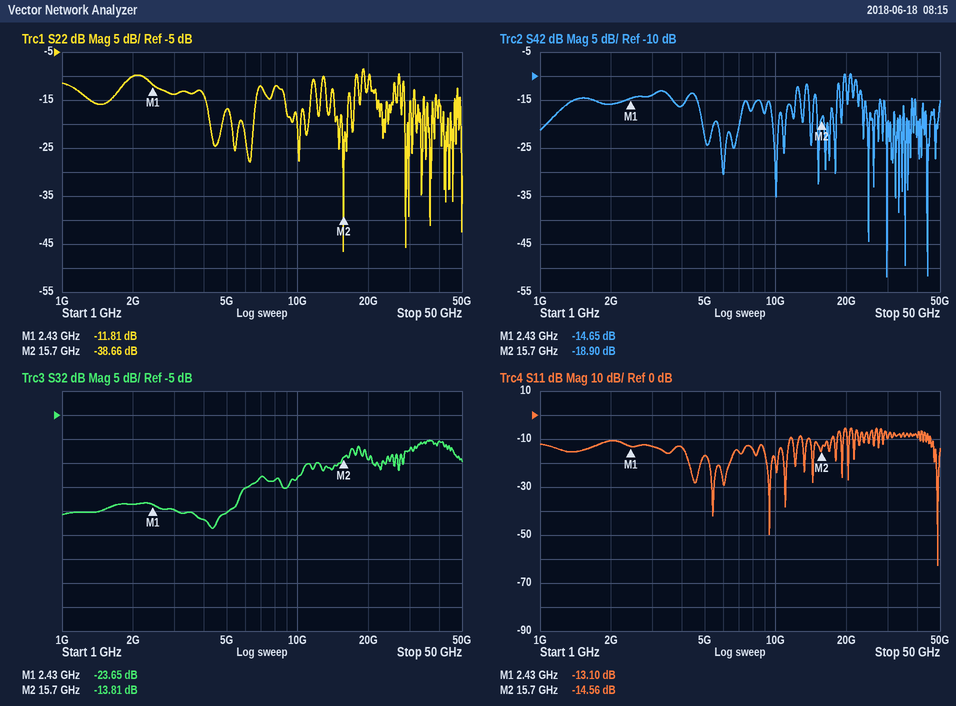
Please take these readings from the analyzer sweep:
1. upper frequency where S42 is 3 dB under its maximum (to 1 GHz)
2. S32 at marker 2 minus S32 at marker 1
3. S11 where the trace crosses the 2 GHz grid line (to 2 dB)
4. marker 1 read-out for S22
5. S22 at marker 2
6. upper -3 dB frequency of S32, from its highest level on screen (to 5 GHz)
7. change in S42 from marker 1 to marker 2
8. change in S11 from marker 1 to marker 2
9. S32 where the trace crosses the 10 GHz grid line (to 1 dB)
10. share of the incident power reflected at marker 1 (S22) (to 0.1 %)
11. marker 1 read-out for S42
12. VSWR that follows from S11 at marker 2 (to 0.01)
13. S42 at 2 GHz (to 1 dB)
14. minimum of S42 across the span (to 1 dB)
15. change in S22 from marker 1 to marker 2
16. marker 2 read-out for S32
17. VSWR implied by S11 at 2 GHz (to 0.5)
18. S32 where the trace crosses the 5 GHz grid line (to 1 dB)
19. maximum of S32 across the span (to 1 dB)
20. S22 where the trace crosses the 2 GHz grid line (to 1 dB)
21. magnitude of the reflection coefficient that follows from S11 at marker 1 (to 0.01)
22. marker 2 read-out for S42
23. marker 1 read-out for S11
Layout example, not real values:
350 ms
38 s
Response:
21 GHz
9.84 dB
-10 dB
-11.81 dB
-38.66 dB
45 GHz
-4.25 dB
-1.46 dB
-18 dB
6.6 %
-14.65 dB
1.46
-16 dB
-52 dB
-26.85 dB
-13.81 dB
2.0
-25 dB
-10 dB
-10 dB
0.22
-18.90 dB
-13.10 dB
